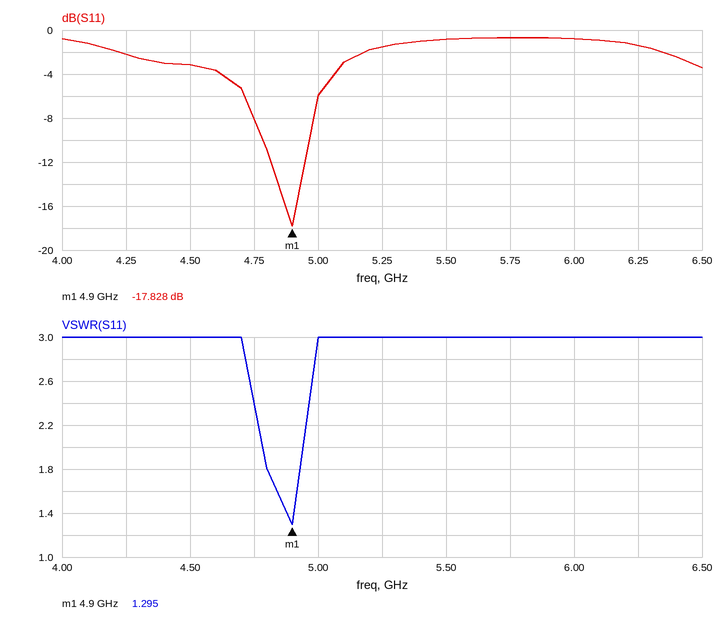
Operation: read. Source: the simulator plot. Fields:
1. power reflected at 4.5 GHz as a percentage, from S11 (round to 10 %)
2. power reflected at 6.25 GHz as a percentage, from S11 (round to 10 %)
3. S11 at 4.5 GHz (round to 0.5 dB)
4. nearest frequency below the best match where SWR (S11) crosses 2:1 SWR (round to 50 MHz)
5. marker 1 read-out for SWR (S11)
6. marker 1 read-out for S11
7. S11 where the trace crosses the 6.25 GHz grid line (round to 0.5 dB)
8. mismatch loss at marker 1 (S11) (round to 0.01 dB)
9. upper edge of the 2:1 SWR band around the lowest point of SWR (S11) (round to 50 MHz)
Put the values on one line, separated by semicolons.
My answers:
50 %; 70 %; -3.0 dB; 4.80 GHz; 1.295; -17.828 dB; -1.5 dB; 0.07 dB; 4.95 GHz
